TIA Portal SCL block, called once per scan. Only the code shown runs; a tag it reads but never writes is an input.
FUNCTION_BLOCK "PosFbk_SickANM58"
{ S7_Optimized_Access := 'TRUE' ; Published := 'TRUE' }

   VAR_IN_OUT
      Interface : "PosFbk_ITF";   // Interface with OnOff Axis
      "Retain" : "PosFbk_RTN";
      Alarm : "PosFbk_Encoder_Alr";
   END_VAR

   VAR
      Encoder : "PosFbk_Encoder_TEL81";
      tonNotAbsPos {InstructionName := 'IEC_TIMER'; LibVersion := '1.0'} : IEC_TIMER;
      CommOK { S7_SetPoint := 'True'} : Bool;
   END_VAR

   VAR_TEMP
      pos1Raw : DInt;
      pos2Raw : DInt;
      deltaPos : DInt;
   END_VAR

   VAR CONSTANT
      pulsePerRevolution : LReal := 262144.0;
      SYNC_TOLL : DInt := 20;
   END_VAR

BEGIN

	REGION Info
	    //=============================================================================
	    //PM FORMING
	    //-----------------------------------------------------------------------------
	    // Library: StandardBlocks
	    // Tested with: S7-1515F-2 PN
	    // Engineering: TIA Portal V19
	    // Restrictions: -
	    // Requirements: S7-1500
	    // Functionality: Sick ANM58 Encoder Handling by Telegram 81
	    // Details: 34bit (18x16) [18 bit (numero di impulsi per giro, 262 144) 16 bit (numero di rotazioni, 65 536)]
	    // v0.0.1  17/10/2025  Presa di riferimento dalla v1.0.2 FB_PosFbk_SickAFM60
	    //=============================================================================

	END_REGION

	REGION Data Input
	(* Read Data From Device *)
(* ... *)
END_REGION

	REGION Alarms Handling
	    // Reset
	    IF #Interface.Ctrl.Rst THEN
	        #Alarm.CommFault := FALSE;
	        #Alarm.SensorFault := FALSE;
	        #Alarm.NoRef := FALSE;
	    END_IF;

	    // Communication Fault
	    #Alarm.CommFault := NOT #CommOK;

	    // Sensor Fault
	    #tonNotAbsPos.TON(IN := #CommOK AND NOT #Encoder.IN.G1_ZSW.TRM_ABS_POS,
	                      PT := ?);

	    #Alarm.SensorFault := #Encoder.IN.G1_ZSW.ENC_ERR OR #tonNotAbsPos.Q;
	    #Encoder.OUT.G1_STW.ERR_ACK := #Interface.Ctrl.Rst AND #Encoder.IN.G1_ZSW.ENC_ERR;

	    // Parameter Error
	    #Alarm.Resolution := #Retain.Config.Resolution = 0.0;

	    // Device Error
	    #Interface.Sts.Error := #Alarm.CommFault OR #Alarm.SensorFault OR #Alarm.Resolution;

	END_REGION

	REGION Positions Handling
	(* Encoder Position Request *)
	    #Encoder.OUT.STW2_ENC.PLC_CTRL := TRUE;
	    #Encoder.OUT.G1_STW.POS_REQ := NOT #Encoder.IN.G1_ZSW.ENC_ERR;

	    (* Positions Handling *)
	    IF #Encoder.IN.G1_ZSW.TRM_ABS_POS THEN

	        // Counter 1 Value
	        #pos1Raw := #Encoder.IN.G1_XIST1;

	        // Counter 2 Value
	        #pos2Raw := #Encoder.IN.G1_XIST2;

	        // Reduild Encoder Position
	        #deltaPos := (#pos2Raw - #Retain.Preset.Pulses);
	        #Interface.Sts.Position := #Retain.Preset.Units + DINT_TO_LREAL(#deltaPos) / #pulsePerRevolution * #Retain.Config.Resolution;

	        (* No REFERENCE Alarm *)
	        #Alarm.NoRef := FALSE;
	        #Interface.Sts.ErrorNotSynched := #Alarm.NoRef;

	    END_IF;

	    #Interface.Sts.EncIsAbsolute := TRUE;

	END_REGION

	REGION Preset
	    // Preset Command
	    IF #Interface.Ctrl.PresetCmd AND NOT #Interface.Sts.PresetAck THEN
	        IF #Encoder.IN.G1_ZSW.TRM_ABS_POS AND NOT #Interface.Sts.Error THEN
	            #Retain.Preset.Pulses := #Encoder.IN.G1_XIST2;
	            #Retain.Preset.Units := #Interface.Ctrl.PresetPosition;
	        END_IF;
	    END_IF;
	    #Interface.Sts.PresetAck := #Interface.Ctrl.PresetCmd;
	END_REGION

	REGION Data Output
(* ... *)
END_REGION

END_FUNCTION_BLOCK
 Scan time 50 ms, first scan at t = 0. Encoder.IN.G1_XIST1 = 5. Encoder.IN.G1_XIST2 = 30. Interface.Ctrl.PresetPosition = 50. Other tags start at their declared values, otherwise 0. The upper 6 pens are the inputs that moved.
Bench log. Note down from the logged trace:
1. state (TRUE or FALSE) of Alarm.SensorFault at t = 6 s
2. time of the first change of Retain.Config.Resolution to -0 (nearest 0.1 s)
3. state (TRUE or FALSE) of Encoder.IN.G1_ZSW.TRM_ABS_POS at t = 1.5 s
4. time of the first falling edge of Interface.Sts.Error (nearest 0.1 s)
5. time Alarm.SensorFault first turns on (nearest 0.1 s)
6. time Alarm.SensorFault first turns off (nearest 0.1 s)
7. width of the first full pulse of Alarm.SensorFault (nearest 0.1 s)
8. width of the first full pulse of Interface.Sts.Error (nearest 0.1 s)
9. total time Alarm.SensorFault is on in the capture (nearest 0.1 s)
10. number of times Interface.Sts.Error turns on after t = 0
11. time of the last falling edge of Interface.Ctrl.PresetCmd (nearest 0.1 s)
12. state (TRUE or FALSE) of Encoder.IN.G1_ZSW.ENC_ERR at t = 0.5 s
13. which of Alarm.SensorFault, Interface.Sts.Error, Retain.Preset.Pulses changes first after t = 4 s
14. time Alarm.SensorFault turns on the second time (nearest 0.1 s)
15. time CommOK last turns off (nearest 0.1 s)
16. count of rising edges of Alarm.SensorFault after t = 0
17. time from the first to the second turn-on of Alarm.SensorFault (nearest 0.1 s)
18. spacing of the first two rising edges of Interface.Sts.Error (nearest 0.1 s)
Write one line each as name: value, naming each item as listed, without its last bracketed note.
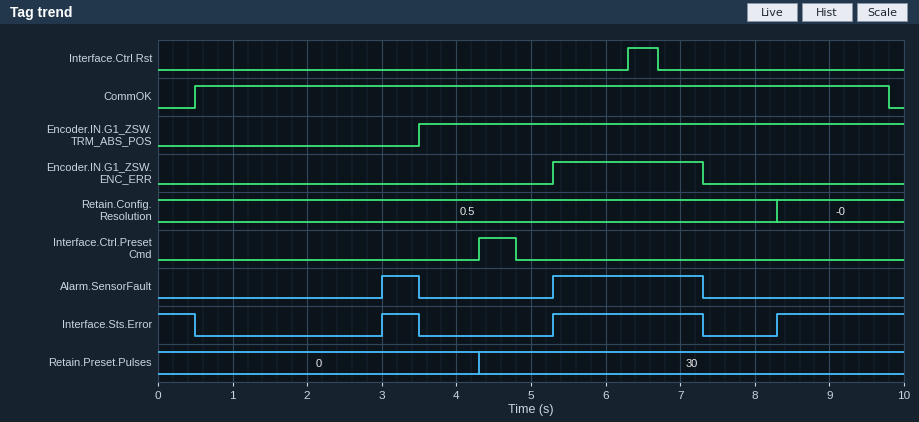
state (TRUE or FALSE) of Alarm.SensorFault at t = 6 s: TRUE
time of the first change of Retain.Config.Resolution to -0: 8.3 s
state (TRUE or FALSE) of Encoder.IN.G1_ZSW.TRM_ABS_POS at t = 1.5 s: FALSE
time of the first falling edge of Interface.Sts.Error: 0.5 s
time Alarm.SensorFault first turns on: 3.0 s
time Alarm.SensorFault first turns off: 3.5 s
width of the first full pulse of Alarm.SensorFault: 0.5 s
width of the first full pulse of Interface.Sts.Error: 0.5 s
total time Alarm.SensorFault is on in the capture: 2.5 s
number of times Interface.Sts.Error turns on after t = 0: 3
time of the last falling edge of Interface.Ctrl.PresetCmd: 4.8 s
state (TRUE or FALSE) of Encoder.IN.G1_ZSW.ENC_ERR at t = 0.5 s: FALSE
which of Alarm.SensorFault, Interface.Sts.Error, Retain.Preset.Pulses changes first after t = 4 s: Retain.Preset.Pulses
time Alarm.SensorFault turns on the second time: 5.3 s
time CommOK last turns off: 9.8 s
count of rising edges of Alarm.SensorFault after t = 0: 2
time from the first to the second turn-on of Alarm.SensorFault: 2.3 s
spacing of the first two rising edges of Interface.Sts.Error: 2.3 s
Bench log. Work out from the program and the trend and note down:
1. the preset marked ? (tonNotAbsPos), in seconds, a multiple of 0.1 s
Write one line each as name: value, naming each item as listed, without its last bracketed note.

the preset marked ? (tonNotAbsPos), in seconds, a multiple of 0.1 s: 2.5 s
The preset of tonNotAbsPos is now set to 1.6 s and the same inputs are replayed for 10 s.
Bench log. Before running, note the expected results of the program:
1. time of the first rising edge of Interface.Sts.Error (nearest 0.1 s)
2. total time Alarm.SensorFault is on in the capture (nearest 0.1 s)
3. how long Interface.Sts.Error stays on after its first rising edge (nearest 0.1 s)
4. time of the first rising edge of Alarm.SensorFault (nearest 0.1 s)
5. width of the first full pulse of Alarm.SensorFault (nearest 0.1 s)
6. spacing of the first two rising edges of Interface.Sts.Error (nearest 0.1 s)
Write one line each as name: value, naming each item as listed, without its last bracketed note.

time of the first rising edge of Interface.Sts.Error: 2.1 s
total time Alarm.SensorFault is on in the capture: 3.4 s
how long Interface.Sts.Error stays on after its first rising edge: 1.4 s
time of the first rising edge of Alarm.SensorFault: 2.1 s
width of the first full pulse of Alarm.SensorFault: 1.4 s
spacing of the first two rising edges of Interface.Sts.Error: 3.2 s
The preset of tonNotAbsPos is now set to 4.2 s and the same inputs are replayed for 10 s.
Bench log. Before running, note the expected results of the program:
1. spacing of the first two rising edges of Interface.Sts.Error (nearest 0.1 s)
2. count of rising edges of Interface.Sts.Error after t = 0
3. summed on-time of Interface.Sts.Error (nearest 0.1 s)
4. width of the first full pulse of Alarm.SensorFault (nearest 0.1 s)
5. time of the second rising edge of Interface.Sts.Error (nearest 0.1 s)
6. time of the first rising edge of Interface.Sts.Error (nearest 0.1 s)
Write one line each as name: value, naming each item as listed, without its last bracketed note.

spacing of the first two rising edges of Interface.Sts.Error: 3.0 s
count of rising edges of Interface.Sts.Error after t = 0: 2
summed on-time of Interface.Sts.Error: 4.2 s
width of the first full pulse of Alarm.SensorFault: 2.0 s
time of the second rising edge of Interface.Sts.Error: 8.3 s
time of the first rising edge of Interface.Sts.Error: 5.3 s
